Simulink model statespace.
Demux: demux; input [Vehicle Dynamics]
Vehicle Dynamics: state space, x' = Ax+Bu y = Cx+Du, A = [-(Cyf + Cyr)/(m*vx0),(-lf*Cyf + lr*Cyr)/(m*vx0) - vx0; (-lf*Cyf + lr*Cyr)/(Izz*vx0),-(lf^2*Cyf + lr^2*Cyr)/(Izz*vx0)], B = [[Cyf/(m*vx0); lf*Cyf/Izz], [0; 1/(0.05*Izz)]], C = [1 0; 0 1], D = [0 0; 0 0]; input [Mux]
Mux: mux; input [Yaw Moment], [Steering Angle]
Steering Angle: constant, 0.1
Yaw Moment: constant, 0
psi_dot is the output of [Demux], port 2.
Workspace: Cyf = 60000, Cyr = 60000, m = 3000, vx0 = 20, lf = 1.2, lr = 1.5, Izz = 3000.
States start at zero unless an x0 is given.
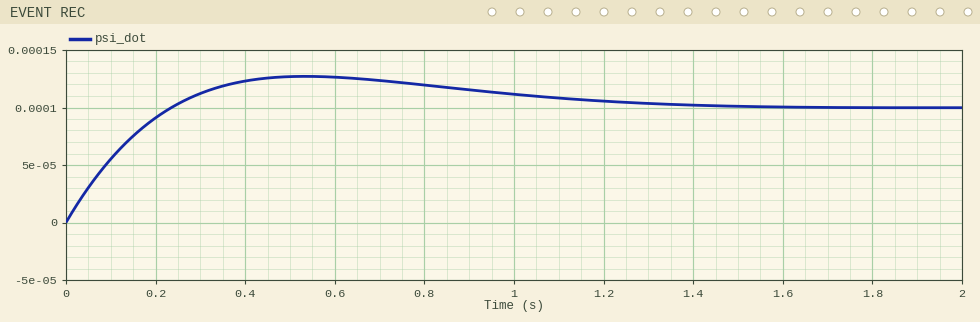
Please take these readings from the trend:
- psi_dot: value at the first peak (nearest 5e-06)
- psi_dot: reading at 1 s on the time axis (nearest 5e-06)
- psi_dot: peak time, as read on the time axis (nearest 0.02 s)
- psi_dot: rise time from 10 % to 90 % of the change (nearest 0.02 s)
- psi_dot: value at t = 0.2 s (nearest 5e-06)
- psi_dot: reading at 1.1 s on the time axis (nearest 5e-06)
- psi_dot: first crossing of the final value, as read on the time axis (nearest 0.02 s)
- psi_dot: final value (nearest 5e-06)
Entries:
0.000125
0.000110
0.54 s
0.18 s
0.000090
0.000110
0.24 s
0.000100
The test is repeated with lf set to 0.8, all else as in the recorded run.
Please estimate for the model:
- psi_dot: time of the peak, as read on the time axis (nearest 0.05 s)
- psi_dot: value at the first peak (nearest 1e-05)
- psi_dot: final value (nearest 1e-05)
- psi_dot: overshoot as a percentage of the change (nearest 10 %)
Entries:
0.40 s
0.00012
0.00007
70 %
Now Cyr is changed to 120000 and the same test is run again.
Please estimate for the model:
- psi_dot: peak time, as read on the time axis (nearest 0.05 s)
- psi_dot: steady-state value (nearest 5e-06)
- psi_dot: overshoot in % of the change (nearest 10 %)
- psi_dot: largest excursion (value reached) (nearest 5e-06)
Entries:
0.25 s
0.000040
70 %
0.000065
